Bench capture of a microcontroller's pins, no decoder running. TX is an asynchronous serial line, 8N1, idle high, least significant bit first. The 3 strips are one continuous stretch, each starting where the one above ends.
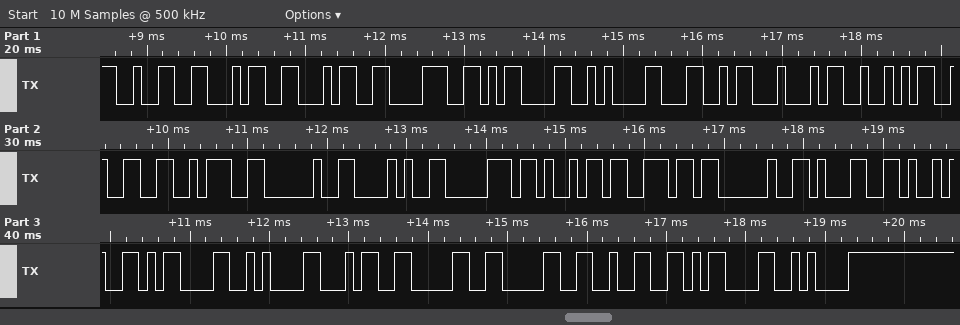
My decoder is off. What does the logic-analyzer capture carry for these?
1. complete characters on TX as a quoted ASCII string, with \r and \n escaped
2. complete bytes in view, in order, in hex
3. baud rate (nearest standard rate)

"2448\r\nLDR2: (pin 1)\r\n4002\r\n"
0x32 0x34 0x34 0x38 0x0D 0x0A 0x4C 0x44 0x52 0x32 0x3A 0x20 0x28 0x70 0x69 0x6E 0x20 0x31 0x29 0x0D 0x0A 0x34 0x30 0x30 0x32 0x0D 0x0A
9600 baud
